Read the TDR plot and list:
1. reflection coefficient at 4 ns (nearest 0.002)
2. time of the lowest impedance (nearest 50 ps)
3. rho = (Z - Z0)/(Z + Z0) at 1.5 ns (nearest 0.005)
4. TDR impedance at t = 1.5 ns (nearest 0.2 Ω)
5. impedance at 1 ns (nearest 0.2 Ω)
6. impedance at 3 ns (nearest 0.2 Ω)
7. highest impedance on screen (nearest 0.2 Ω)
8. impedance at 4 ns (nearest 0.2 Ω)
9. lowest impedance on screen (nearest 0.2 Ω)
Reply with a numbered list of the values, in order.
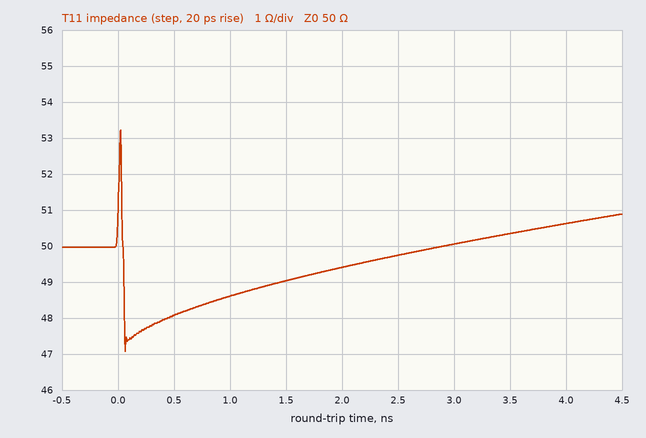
1. +0.006
2. 50 ps
3. -0.010
4. 49.0 Ω
5. 48.6 Ω
6. 50.0 Ω
7. 53.2 Ω
8. 50.6 Ω
9. 47.0 Ω
